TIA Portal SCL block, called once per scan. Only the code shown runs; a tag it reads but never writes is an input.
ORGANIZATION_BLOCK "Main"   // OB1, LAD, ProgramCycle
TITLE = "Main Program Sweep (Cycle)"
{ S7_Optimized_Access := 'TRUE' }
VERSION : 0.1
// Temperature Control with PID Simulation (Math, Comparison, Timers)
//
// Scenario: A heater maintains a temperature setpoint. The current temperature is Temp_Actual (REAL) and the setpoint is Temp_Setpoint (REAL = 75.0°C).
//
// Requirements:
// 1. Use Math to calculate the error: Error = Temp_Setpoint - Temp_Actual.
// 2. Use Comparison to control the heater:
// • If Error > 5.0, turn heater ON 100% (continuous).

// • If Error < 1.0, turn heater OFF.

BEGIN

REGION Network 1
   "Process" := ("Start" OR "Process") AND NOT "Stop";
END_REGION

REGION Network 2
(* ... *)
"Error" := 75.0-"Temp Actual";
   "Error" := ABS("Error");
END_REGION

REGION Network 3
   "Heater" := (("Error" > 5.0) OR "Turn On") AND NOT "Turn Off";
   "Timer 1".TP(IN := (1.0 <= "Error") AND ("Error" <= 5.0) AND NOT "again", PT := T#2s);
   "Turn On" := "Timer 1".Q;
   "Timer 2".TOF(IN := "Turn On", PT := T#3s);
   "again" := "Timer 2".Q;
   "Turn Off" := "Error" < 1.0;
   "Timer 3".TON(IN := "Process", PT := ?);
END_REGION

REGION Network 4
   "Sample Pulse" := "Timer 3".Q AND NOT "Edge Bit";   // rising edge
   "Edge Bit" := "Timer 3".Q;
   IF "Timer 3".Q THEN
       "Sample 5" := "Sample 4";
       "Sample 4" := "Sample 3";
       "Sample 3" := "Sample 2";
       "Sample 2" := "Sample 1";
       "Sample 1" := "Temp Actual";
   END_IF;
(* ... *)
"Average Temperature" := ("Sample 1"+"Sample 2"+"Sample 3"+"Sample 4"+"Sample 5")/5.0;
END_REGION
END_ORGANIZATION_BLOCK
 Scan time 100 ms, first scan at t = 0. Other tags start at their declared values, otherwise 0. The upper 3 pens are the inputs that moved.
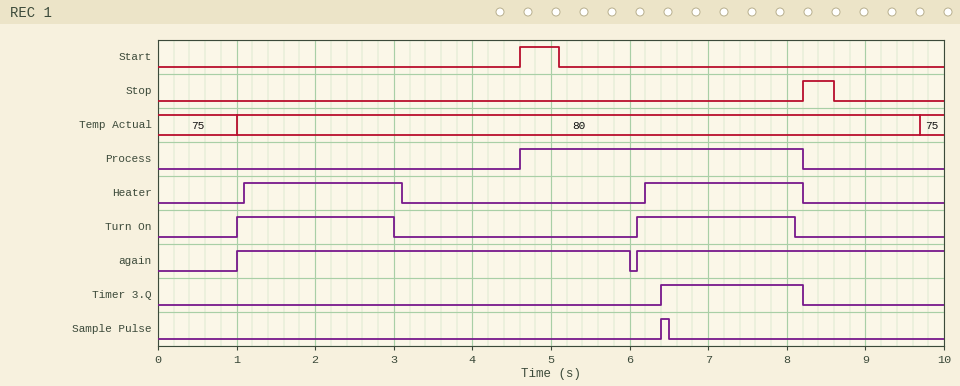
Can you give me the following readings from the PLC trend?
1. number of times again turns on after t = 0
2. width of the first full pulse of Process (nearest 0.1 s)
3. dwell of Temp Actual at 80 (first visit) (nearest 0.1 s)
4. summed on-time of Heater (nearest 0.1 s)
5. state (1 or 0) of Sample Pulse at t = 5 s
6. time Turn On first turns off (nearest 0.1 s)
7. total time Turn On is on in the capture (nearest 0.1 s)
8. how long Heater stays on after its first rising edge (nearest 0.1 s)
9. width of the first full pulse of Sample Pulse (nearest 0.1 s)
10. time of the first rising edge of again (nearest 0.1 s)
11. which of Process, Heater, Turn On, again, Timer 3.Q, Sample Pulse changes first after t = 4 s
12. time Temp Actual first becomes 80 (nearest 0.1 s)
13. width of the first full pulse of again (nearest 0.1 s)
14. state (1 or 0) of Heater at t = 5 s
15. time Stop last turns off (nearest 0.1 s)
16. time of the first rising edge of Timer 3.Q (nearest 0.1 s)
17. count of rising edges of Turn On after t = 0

2
3.6 s
8.7 s
4.0 s
0
3.0 s
4.0 s
2.0 s
0.1 s
1.0 s
Process
1.0 s
5.0 s
0
8.6 s
6.4 s
2
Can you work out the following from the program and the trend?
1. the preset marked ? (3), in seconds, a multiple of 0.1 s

1.8 s
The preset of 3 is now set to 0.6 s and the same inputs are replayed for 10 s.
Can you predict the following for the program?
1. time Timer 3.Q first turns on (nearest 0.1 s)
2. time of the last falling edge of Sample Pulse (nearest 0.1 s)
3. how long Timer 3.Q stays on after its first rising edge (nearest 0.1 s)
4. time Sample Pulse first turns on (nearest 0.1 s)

5.2 s
5.3 s
3.0 s
5.2 s
